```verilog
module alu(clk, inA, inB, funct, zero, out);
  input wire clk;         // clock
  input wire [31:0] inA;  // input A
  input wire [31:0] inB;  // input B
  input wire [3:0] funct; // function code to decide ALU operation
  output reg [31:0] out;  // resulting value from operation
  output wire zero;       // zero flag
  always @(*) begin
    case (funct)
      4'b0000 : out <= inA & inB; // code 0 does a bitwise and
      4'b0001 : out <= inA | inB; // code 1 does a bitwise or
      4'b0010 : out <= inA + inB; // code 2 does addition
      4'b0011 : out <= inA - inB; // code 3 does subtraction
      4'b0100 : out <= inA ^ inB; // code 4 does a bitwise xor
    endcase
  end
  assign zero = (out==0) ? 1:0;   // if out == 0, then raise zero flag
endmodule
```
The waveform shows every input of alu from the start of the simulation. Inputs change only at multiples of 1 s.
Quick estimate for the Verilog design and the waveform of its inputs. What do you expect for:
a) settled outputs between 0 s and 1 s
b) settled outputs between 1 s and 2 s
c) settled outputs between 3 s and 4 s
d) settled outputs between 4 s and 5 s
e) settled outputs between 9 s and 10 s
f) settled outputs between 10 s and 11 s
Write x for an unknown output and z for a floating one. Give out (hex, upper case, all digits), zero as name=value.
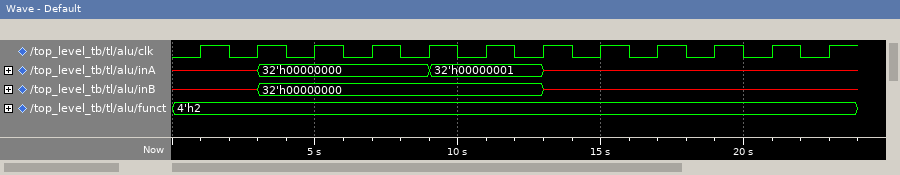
out=x, zero=x
out=x, zero=x
out=00000000, zero=1
out=00000000, zero=1
out=00000001, zero=0
out=00000001, zero=0
